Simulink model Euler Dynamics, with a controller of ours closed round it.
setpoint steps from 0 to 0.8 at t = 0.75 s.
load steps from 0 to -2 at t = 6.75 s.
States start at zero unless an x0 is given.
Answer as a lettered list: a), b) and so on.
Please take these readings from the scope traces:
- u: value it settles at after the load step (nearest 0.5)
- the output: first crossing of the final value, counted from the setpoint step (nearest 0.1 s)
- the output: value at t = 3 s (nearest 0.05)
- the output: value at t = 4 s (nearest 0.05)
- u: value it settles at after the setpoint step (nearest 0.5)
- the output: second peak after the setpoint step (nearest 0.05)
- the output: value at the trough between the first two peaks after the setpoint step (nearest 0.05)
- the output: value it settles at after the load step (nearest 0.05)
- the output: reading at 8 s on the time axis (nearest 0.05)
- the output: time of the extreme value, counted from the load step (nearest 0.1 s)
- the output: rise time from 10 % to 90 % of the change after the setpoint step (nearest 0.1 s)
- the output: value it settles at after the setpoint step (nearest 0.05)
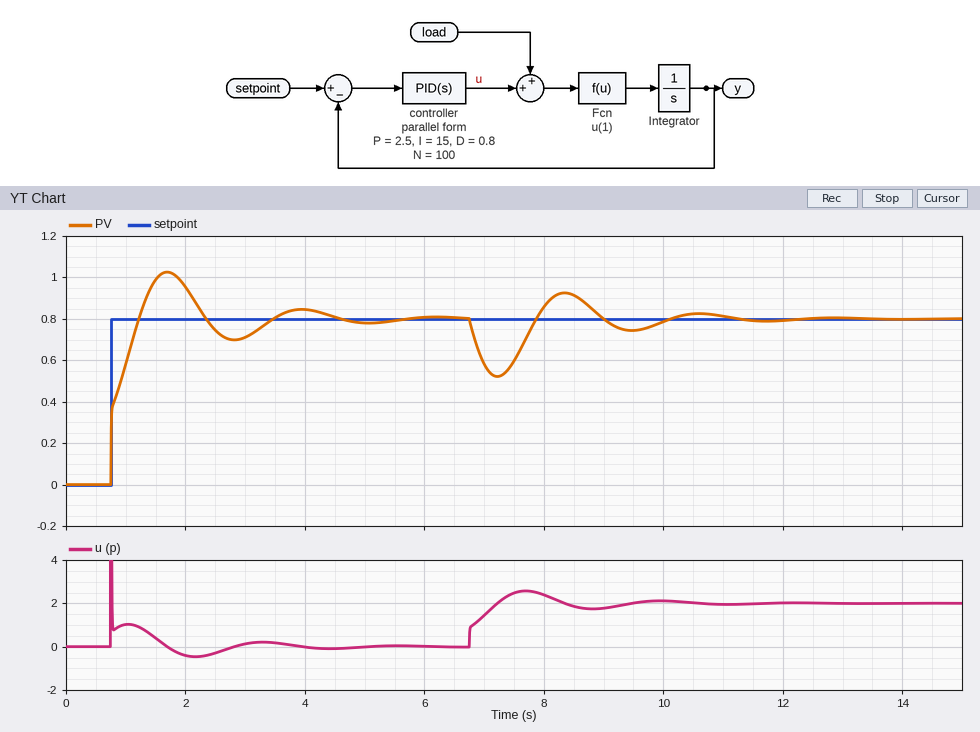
a) 2.0
b) 0.5 s
c) 0.70
d) 0.85
e) 0.0
f) 0.85
g) 0.70
h) 0.80
i) 0.85
j) 0.5 s
k) 0.4 s
l) 0.80
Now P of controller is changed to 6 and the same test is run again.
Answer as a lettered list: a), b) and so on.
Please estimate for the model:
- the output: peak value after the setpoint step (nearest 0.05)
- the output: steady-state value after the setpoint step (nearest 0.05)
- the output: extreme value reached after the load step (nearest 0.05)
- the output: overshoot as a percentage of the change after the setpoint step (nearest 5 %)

a) 0.90
b) 0.80
c) 0.60
d) 15 %
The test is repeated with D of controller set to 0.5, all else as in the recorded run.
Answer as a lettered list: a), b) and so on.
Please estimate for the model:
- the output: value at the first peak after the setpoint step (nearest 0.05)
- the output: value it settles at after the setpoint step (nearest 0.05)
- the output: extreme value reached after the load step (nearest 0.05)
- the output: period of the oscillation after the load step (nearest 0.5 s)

a) 1.05
b) 0.80
c) 0.50
d) 2.0 s
